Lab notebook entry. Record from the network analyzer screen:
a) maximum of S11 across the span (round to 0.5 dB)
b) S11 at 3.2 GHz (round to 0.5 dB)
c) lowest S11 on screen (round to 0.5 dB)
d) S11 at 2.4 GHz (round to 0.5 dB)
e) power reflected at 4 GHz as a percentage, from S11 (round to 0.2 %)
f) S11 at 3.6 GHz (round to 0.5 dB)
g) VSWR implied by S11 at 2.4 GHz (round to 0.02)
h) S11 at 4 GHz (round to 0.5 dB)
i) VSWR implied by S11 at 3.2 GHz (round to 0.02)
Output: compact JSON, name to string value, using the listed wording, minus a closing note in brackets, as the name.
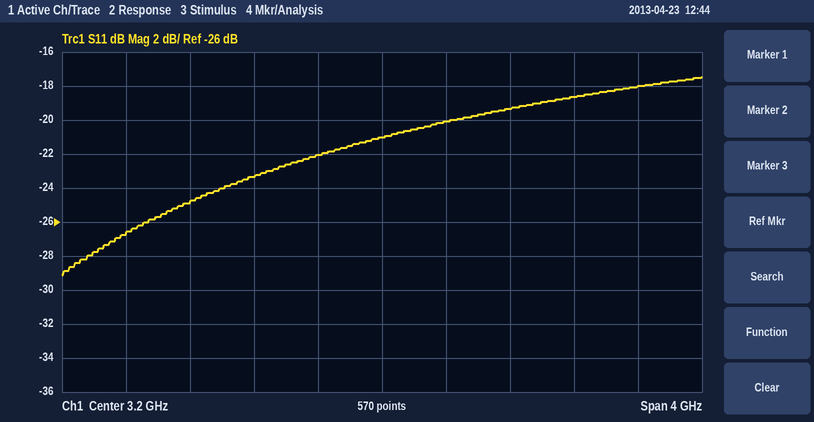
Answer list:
{"maximum of S11 across the span": "-17.5 dB", "S11 at 3.2 GHz": "-21.0 dB", "lowest S11 on screen": "-29.0 dB", "S11 at 2.4 GHz": "-23.5 dB", "power reflected at 4 GHz as a percentage, from S11": "1.2 %", "S11 at 3.6 GHz": "-20.0 dB", "VSWR implied by S11 at 2.4 GHz": "1.14", "S11 at 4 GHz": "-19.5 dB", "VSWR implied by S11 at 3.2 GHz": "1.20"}
